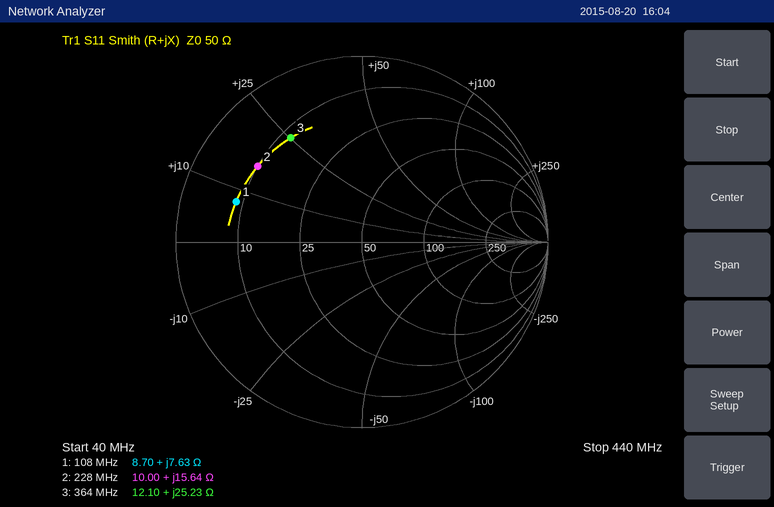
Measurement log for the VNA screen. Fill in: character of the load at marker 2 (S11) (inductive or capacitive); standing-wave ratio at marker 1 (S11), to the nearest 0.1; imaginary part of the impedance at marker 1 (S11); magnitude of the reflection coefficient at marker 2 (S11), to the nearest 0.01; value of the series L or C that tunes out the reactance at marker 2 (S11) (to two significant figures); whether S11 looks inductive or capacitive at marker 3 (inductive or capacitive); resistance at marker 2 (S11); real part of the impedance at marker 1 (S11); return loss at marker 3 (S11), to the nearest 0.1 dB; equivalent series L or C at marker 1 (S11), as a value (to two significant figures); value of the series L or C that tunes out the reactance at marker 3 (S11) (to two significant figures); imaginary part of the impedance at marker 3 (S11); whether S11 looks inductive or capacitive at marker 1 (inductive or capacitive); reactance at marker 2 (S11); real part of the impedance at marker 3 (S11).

inductive
5.9
+7.63 Ω
0.69
45 pF
inductive
10.00 Ω
8.70 Ω
3.4 dB
11 nH
17 pF
+25.23 Ω
inductive
+15.64 Ω
12.10 Ω
